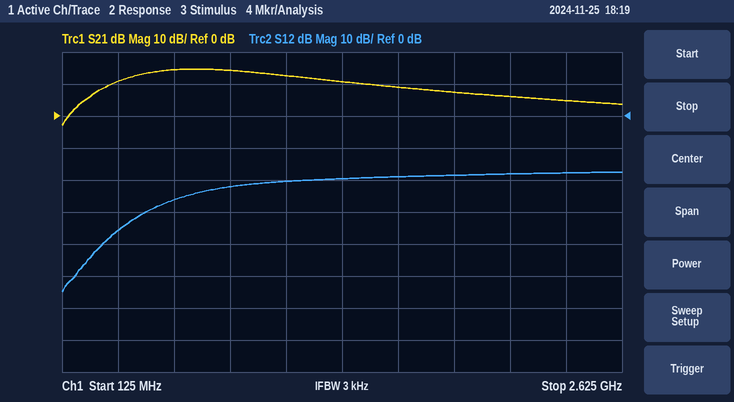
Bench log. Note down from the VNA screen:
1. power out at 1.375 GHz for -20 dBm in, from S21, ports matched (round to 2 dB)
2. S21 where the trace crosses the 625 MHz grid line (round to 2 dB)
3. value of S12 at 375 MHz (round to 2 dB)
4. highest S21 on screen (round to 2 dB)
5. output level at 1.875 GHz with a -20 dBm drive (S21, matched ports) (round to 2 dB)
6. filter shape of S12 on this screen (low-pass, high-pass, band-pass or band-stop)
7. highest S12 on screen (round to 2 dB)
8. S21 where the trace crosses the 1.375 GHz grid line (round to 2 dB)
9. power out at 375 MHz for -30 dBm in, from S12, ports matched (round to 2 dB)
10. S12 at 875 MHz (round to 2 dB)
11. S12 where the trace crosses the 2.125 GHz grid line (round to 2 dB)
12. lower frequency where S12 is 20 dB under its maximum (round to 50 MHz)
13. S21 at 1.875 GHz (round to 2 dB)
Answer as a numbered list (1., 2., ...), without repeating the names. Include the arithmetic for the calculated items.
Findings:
1. -20 dBm + (10 dB) = -10 dBm
2. 14 dB
3. -36 dB
4. 14 dB
5. -20 dBm + (8 dB) = -12 dBm
6. high-pass
7. -18 dB
8. 10 dB
9. -30 dBm + (-36 dB) = -66 dBm
10. -22 dB
11. -18 dB
12. 350 MHz
13. 8 dB
